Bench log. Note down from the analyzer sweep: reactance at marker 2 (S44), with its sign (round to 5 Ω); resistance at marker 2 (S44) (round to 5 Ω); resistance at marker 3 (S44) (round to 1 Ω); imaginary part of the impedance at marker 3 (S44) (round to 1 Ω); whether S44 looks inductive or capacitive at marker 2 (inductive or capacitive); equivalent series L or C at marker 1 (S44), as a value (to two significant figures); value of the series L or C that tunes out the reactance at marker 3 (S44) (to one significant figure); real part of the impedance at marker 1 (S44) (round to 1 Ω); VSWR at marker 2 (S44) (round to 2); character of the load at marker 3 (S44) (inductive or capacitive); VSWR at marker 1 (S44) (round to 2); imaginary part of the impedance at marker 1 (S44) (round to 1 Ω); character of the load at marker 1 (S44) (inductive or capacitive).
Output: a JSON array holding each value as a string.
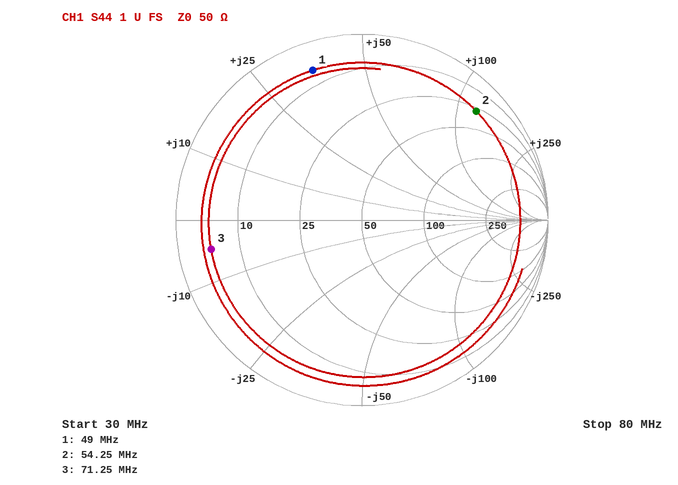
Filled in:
["+120 Ω", "30 Ω", "5 Ω", "-5 Ω", "inductive", "120 nH", "10 nH", "6 Ω", "12", "capacitive", "12", "+36 Ω", "inductive"]
